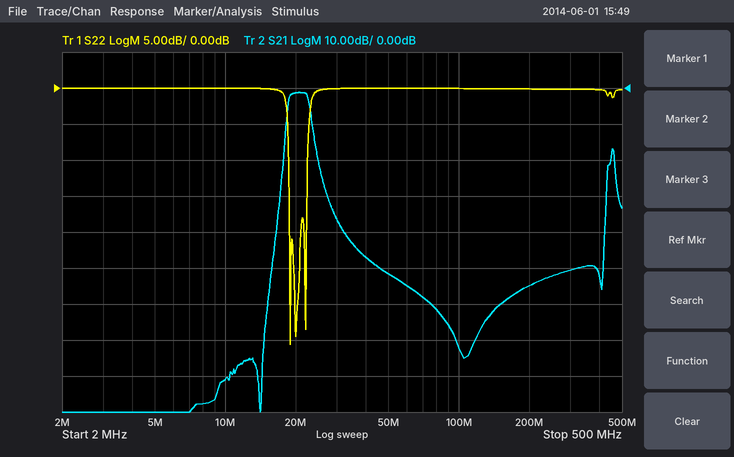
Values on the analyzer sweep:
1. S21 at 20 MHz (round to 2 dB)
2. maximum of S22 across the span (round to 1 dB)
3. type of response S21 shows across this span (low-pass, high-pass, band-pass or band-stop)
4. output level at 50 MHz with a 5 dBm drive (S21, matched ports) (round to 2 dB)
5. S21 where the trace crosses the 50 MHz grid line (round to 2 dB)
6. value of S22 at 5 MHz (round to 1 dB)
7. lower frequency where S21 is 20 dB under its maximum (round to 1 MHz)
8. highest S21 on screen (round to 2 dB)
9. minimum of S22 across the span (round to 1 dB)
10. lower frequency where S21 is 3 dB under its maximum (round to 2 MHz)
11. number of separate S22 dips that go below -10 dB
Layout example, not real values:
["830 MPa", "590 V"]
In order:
["-2 dB", "0 dB", "band-pass", "-46 dBm", "-52 dB", "0 dB", "18 MHz", "-2 dB", "-36 dB", "18 MHz", "3"]
